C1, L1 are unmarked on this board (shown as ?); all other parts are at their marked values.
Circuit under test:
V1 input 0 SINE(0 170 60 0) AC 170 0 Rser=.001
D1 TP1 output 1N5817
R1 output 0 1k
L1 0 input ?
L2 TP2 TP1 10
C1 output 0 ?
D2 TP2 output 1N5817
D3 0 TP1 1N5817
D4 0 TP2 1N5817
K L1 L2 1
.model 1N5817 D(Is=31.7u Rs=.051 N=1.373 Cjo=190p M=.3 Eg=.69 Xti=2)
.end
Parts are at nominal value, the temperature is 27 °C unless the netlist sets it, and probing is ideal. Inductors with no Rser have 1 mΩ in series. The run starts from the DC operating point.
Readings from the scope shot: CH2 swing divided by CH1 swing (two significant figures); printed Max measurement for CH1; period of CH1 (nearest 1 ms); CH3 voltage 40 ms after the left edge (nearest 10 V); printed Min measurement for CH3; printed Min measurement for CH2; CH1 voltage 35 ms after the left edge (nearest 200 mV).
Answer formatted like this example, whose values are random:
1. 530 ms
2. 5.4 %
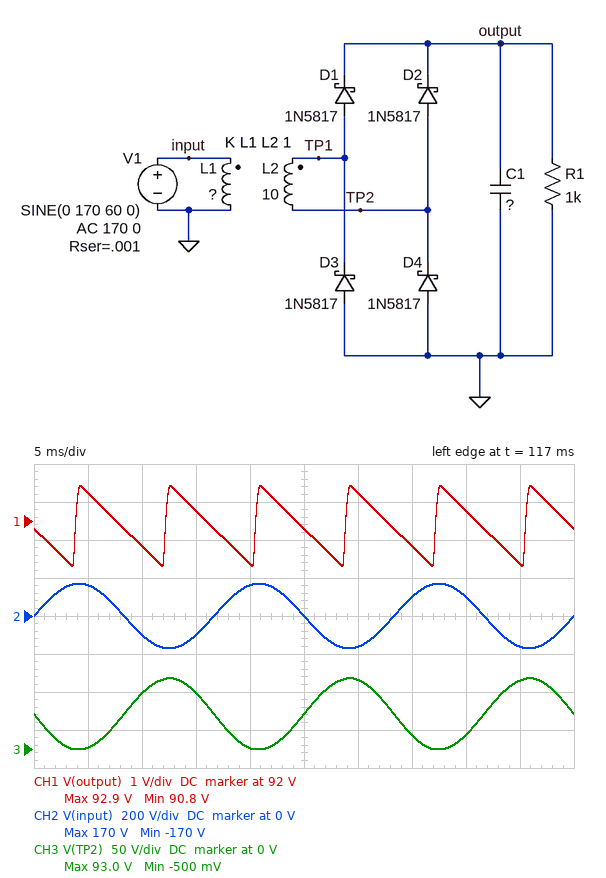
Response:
1. 160
2. 92.9 V
3. 8 ms
4. 20 V
5. -500 mV
6. -170 V
7. 91.4 V
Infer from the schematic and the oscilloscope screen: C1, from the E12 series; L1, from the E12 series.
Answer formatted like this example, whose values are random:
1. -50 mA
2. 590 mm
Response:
1. 330 µF
2. 33 H
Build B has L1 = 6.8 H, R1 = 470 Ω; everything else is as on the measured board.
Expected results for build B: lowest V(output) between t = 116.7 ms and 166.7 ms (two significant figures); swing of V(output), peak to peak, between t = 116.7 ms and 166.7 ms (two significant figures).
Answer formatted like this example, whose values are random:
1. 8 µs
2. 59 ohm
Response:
1. 200 V
2. 9.6 V
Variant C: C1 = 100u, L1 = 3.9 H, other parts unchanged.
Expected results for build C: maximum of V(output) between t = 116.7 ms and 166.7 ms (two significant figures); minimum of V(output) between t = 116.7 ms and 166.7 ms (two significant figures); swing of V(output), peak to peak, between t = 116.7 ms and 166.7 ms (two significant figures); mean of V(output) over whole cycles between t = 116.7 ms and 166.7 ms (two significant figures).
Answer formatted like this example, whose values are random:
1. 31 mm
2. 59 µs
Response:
1. 270 V
2. 250 V
3. 19 V
4. 260 V
